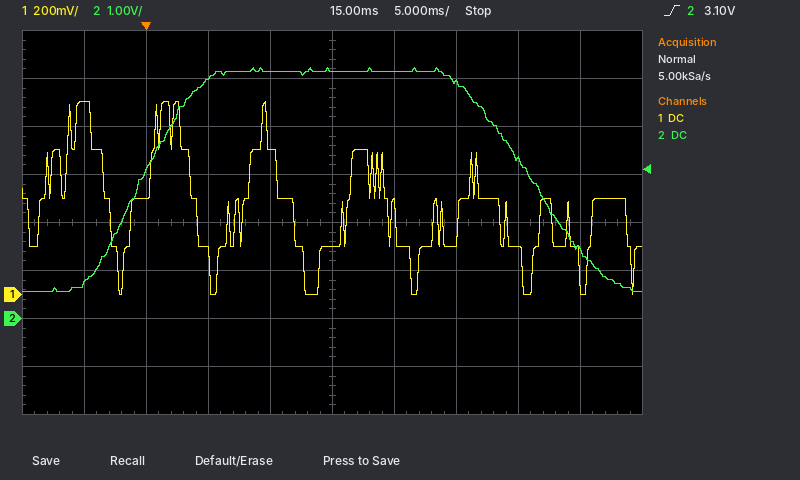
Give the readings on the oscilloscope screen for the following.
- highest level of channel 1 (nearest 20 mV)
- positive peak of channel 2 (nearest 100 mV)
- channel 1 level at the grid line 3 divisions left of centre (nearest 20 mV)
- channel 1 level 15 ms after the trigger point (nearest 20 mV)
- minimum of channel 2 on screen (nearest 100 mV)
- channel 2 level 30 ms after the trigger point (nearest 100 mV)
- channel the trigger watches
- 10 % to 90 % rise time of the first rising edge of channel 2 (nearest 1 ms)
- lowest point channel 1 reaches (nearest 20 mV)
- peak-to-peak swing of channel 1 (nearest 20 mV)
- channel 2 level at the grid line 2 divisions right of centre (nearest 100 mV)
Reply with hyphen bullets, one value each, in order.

- 800 mV
- 5.2 V
- 400 mV
- 200 mV
- 600 mV
- 3.3 V
- channel 2
- 8 ms
- 0 mV
- 800 mV
- 4.9 V
